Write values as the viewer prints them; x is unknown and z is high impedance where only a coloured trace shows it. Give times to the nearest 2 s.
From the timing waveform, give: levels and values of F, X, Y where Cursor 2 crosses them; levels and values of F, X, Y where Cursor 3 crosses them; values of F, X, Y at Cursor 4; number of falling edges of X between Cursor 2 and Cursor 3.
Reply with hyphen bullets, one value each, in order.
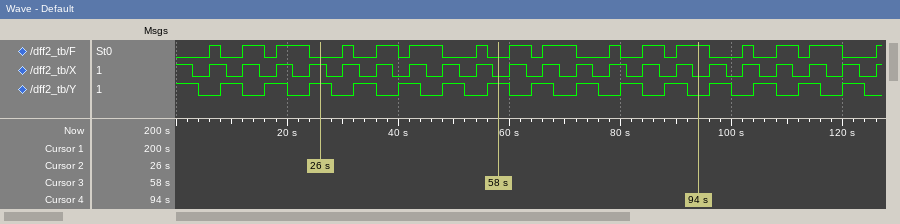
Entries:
- F=0, X=1, Y=1
- F=0, X=0, Y=1
- F=1, X=0, Y=0
- 6
